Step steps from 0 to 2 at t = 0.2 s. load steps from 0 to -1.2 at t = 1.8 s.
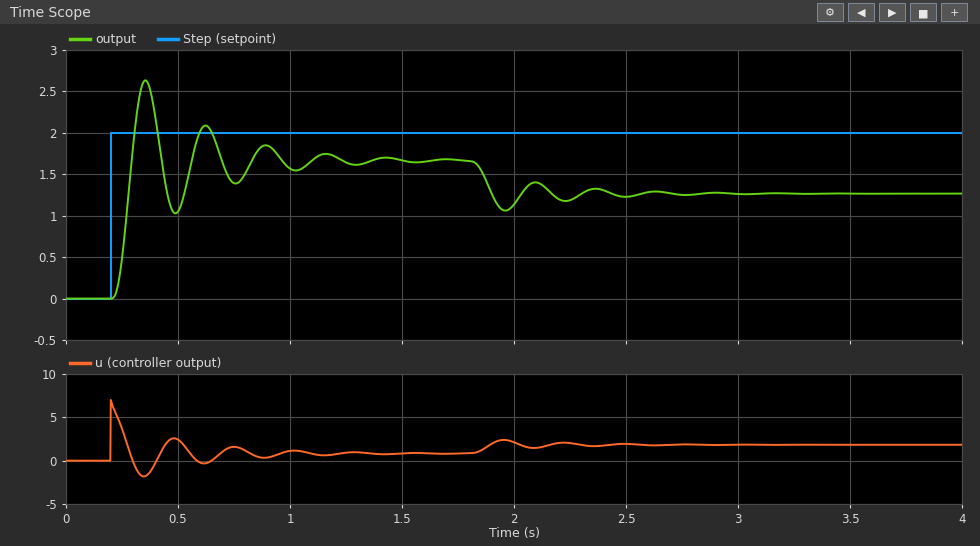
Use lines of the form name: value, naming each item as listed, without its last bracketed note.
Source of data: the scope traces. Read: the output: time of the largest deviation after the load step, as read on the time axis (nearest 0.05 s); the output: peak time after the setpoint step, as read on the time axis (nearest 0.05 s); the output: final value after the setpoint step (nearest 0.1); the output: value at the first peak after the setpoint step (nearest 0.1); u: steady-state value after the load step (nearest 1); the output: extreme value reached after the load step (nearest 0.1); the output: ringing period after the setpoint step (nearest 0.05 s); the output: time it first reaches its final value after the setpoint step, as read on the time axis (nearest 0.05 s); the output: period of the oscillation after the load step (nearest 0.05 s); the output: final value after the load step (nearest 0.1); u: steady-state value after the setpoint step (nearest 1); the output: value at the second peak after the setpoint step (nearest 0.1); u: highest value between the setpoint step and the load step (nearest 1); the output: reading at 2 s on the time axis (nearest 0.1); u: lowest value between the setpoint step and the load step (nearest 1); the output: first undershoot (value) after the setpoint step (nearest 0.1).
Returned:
the output: time of the largest deviation after the load step, as read on the time axis: 1.95 s
the output: peak time after the setpoint step, as read on the time axis: 0.35 s
the output: final value after the setpoint step: 1.7
the output: value at the first peak after the setpoint step: 2.6
u: steady-state value after the load step: 2
the output: extreme value reached after the load step: 1.1
the output: ringing period after the setpoint step: 0.25 s
the output: time it first reaches its final value after the setpoint step, as read on the time axis: 0.30 s
the output: period of the oscillation after the load step: 0.25 s
the output: final value after the load step: 1.3
u: steady-state value after the setpoint step: 1
the output: value at the second peak after the setpoint step: 2.1
u: highest value between the setpoint step and the load step: 7
the output: reading at 2 s on the time axis: 1.1
u: lowest value between the setpoint step and the load step: -2
the output: first undershoot (value) after the setpoint step: 1.0
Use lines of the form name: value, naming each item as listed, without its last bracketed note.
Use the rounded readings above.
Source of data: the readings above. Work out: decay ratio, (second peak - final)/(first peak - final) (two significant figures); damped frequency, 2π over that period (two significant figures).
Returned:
decay ratio, (second peak - final)/(first peak - final): 0.44
damped frequency, 2π over that period: 25 rad/s
